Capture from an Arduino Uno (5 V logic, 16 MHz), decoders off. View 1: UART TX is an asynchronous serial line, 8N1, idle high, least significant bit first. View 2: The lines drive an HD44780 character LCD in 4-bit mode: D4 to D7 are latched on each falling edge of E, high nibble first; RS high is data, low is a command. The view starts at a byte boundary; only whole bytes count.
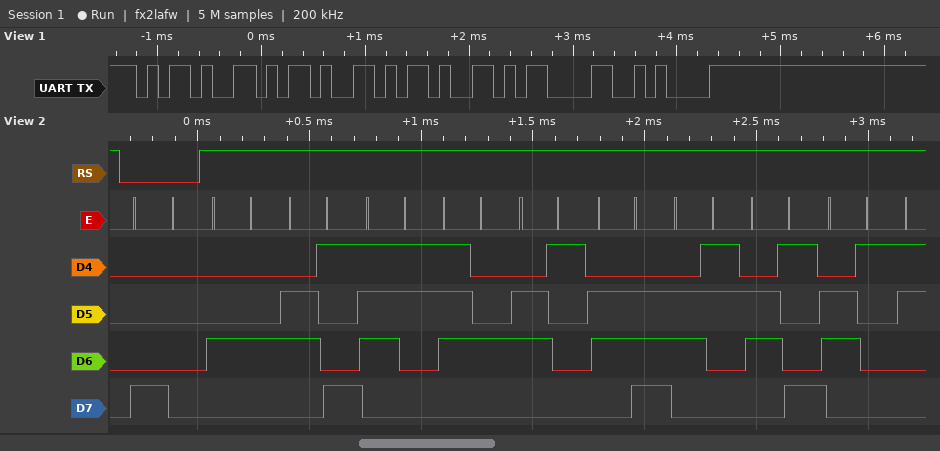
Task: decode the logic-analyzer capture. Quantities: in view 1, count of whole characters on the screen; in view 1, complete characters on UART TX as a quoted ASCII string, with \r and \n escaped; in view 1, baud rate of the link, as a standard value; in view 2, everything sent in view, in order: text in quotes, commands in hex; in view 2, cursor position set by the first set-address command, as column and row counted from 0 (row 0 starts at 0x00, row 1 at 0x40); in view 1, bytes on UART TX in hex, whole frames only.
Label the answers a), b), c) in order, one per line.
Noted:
a) 5
b) "---\r\n"
c) 9600 baud
d) 0x80 "Distancia"
e) column 0, row 0
f) 2D 2D 2D 0D 0A
